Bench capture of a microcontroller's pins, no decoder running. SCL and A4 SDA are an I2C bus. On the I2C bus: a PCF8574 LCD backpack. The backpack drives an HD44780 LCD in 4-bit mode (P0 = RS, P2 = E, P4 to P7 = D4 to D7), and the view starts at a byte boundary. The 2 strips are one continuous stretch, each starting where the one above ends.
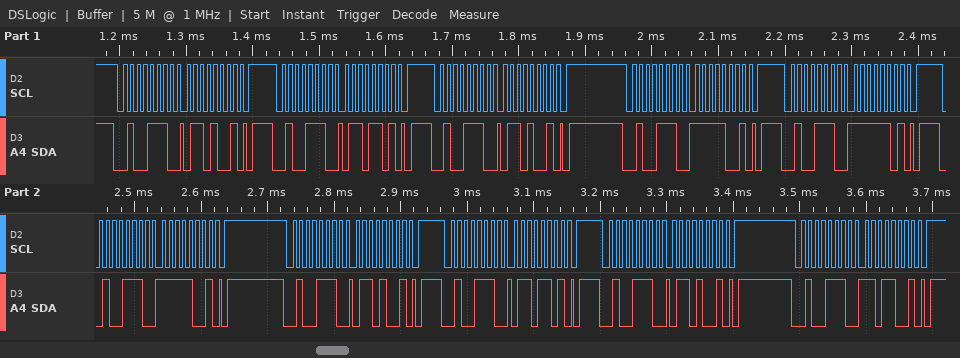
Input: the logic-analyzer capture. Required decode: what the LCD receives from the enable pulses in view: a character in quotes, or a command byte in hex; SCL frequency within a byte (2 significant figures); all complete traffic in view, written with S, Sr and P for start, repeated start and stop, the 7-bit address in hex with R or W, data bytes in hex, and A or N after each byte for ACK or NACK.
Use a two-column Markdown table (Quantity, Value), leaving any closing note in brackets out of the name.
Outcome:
| Quantity | Value |
|---|---|
| what the LCD receives from the enable pulses in view: a character in quotes, or a command byte in hex | 'o' |
| SCL frequency within a byte | 100 kHz |
| all complete traffic in view, written with S, Sr and P for start, repeated start and stop, the 7-bit address in hex with R or W, data bytes in hex, and A or N after each byte for ACK or NACK | S 27W A 69 A P S 27W A 6D A P S 27W A 69 A P S 27W A F9 A P S 27W A FD A P S 27W A F9 A P S 27W A 69 A P S 27W A 6D A P S 27W A 69 A P S 27W A D9 A P |
